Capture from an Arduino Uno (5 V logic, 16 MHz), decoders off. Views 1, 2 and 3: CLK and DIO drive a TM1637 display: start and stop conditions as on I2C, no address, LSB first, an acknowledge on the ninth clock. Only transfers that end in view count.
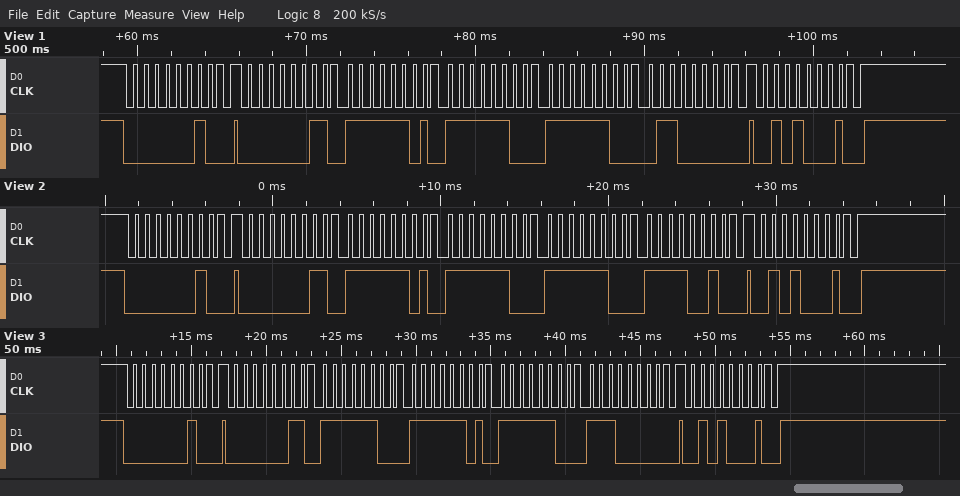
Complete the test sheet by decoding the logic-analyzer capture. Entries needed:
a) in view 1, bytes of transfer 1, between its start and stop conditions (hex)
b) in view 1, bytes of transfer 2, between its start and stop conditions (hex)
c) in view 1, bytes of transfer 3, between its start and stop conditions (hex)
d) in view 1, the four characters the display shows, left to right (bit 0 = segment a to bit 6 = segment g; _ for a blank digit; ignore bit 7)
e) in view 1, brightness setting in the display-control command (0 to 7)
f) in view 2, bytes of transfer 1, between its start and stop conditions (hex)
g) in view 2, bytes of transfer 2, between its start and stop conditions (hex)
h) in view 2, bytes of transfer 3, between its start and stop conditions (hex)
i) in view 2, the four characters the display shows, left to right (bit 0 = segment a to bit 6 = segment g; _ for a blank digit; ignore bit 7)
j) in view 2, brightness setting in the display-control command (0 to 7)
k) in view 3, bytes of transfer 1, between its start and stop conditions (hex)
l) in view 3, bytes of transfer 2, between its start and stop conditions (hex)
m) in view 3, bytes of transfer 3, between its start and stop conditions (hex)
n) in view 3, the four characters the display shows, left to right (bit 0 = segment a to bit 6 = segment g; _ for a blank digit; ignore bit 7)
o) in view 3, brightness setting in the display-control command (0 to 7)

40
C0 BF 3F 3F 06
8A
0001
2
40
C0 BF 3F 3F 4F
8A
0003
2
40
C0 3F BF 3F 07
8A
0007
2
